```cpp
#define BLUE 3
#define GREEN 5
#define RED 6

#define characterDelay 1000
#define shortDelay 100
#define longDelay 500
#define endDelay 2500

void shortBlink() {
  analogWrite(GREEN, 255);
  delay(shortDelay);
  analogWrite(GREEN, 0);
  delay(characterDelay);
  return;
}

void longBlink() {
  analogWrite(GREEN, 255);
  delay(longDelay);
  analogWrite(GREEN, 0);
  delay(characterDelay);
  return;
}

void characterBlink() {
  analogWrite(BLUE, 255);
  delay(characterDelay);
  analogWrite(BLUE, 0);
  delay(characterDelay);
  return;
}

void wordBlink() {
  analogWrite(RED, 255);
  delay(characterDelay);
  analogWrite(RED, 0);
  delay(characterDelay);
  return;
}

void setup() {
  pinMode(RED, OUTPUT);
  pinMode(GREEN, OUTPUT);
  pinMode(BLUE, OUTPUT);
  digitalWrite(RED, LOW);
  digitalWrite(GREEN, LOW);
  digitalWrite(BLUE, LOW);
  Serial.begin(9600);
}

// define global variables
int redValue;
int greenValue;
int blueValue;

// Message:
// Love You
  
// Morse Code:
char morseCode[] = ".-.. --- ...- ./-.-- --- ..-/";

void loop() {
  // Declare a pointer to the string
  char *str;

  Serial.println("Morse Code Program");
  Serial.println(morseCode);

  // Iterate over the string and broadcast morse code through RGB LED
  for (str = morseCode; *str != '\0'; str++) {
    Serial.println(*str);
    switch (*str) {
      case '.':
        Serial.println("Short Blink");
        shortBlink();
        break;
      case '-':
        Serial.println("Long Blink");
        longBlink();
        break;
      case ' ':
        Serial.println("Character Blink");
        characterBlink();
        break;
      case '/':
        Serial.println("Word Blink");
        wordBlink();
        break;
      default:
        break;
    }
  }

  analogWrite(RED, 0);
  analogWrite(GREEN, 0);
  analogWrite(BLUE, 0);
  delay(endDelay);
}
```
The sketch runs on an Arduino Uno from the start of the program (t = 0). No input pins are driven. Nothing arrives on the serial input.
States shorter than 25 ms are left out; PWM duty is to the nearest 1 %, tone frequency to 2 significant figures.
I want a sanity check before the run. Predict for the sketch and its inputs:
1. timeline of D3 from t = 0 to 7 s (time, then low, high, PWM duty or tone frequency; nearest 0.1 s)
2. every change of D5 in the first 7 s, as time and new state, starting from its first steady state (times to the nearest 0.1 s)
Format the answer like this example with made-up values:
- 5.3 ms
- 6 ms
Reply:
- 0 s low; 4.8 s high; 5.8 s low
- 0 s high; 0.1 s low; 1.1 s high; 1.6 s low; 2.6 s high; 2.7 s low; 3.7 s high; 3.8 s low; 6.8 s high
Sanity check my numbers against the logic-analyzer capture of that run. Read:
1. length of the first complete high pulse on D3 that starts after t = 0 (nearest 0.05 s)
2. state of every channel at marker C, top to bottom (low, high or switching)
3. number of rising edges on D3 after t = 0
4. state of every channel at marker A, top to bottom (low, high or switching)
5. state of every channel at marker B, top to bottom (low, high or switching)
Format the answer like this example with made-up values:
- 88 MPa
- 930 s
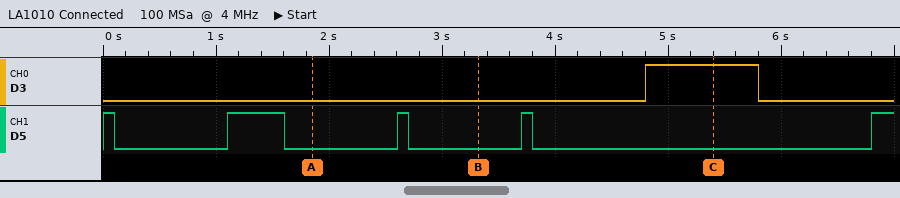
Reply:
- 1.00 s
- D3 high, D5 low
- 1
- D3 low, D5 low
- D3 low, D5 low
